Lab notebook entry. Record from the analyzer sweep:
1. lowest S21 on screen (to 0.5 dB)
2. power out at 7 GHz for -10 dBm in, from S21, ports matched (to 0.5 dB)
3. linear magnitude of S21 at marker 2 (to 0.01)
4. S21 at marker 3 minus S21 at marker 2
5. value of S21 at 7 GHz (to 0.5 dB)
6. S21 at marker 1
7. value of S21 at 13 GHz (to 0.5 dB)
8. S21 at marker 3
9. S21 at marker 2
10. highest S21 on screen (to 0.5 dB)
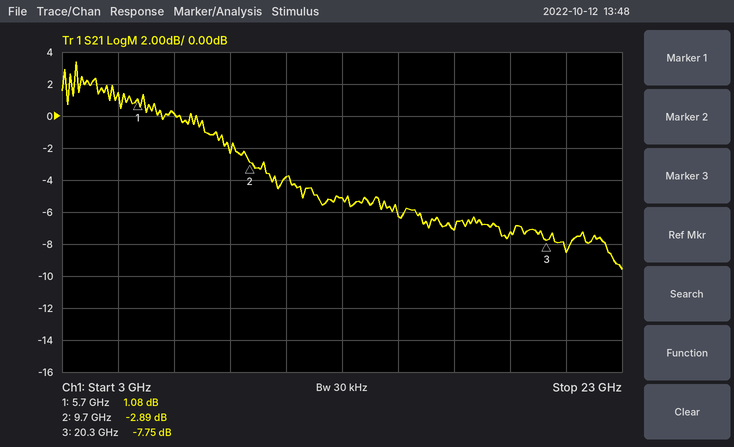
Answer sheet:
-9.5 dB
-10.0 dBm
0.72
-4.86 dB
0.0 dB
1.08 dB
-5.0 dB
-7.75 dB
-2.89 dB
3.5 dB
